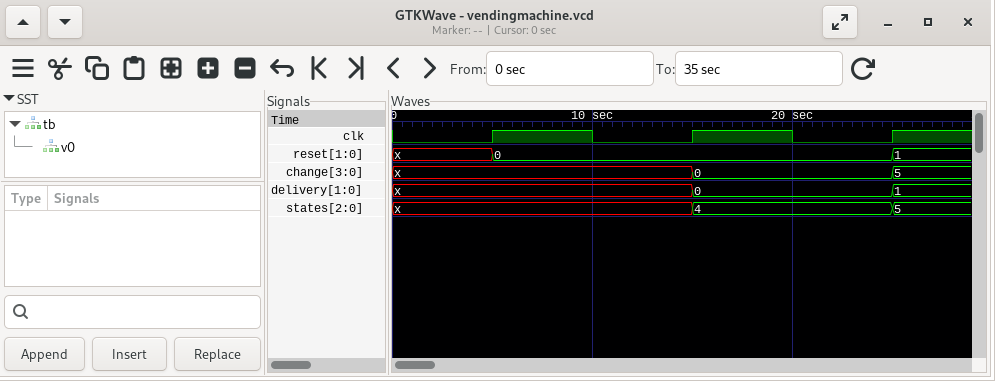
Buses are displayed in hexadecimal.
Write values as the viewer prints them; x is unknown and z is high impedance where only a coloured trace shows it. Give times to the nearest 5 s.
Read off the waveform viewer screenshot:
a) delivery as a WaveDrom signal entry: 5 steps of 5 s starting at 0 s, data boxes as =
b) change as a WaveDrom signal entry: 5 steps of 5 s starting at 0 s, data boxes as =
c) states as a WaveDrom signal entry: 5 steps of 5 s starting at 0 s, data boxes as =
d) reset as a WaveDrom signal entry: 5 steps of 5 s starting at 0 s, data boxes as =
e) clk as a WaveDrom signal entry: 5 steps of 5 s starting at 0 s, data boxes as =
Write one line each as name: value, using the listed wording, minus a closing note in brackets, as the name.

delivery as a WaveDrom signal entry: 5 steps of 5 s starting at 0 s, data boxes as =: {name: 'delivery', wave: 'x..=.', data: '0'}
change as a WaveDrom signal entry: 5 steps of 5 s starting at 0 s, data boxes as =: {name: 'change', wave: 'x..=.', data: '0'}
states as a WaveDrom signal entry: 5 steps of 5 s starting at 0 s, data boxes as =: {name: 'states', wave: 'x..=.', data: '4'}
reset as a WaveDrom signal entry: 5 steps of 5 s starting at 0 s, data boxes as =: {name: 'reset', wave: 'x=...', data: '0'}
clk as a WaveDrom signal entry: 5 steps of 5 s starting at 0 s, data boxes as =: {name: 'clk', wave: '01010'}
